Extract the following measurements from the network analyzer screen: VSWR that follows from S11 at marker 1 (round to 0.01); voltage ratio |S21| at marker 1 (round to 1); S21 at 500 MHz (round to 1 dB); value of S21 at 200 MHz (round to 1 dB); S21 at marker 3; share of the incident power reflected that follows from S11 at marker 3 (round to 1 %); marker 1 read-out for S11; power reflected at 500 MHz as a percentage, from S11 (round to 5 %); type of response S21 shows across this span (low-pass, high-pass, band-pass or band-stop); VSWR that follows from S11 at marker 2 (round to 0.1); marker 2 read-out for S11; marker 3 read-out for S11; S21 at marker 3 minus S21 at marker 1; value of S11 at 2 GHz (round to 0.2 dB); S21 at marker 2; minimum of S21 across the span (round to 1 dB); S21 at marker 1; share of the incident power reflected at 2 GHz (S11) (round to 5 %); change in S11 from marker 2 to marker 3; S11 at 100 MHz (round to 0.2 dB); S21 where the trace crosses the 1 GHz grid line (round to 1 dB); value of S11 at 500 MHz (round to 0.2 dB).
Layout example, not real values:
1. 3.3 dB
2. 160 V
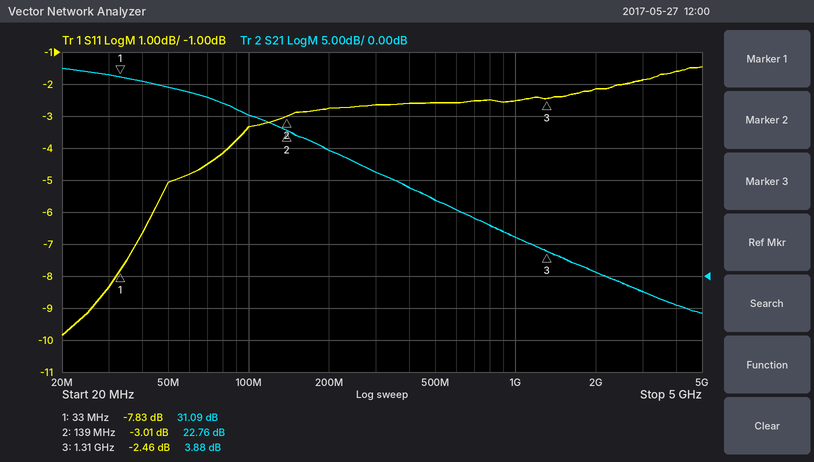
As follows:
1. 2.37
2. 36
3. 12 dB
4. 20 dB
5. 3.88 dB
6. 57 %
7. -7.83 dB
8. 55 %
9. low-pass
10. 5.8
11. -3.01 dB
12. -2.46 dB
13. -27.21 dB
14. -2.2 dB
15. 22.76 dB
16. -6 dB
17. 31.09 dB
18. 60 %
19. 0.55 dB
20. -3.4 dB
21. 6 dB
22. -2.6 dB
